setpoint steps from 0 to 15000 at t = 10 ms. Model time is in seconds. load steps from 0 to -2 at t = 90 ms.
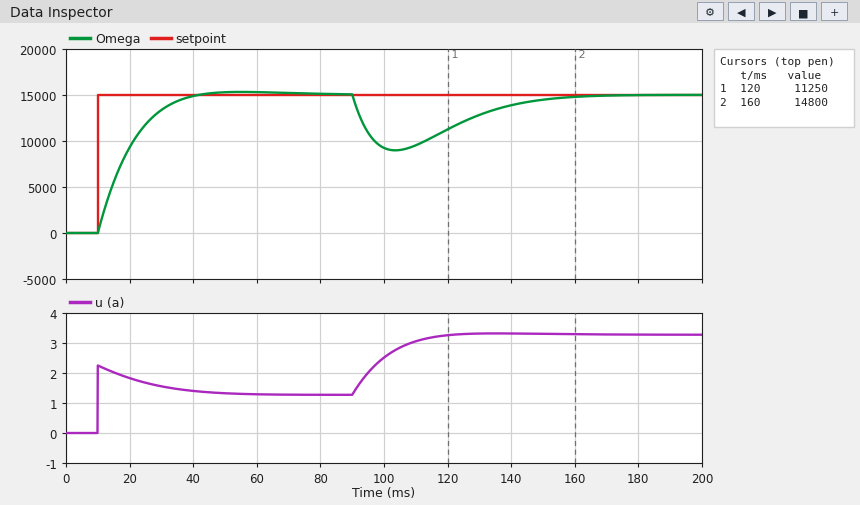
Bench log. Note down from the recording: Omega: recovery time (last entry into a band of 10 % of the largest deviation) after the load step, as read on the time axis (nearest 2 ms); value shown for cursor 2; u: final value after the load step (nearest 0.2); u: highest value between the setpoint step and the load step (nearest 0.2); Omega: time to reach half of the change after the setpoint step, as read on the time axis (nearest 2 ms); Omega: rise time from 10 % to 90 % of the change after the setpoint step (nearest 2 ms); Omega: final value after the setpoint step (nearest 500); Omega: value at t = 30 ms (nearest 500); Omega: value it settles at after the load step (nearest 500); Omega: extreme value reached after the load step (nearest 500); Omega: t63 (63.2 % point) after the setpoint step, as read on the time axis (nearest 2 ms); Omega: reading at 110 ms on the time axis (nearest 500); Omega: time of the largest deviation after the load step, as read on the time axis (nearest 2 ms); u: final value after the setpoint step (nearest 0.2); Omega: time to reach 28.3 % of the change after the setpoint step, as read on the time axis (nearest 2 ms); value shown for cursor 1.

148 ms
14800
3.2
2.2
18 ms
20 ms
15000
13500
15000
9000
20 ms
9500
104 ms
1.2
14 ms
11250
